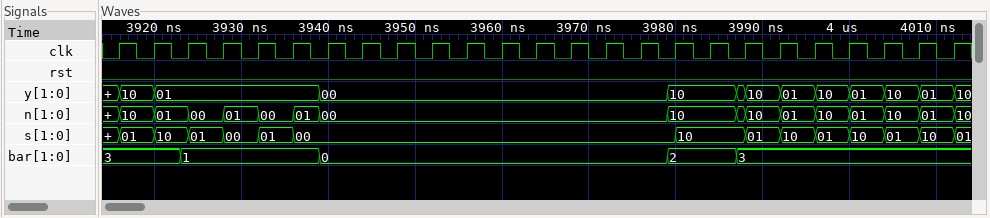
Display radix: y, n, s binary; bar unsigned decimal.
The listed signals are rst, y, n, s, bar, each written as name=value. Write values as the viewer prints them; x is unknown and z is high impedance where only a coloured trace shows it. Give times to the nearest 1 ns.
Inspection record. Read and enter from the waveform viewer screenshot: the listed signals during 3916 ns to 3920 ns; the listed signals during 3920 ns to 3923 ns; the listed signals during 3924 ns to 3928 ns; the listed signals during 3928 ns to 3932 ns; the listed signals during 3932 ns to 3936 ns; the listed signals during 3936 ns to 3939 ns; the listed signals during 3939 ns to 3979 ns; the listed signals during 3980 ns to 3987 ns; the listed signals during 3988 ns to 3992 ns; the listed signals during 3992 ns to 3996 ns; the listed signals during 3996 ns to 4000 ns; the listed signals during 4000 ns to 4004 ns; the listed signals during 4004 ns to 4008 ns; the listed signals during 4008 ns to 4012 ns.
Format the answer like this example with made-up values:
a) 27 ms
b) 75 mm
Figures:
a) rst=0, y=10, n=10, s=01, bar=3
b) rst=0, y=01, n=01, s=10, bar=3
c) rst=0, y=01, n=00, s=01, bar=1
d) rst=0, y=01, n=01, s=00, bar=1
e) rst=0, y=01, n=00, s=01, bar=1
f) rst=0, y=01, n=01, s=00, bar=1
g) rst=0, y=00, n=00, s=00, bar=0
h) rst=0, y=10, n=10, s=10, bar=2
i) rst=0, y=10, n=10, s=01, bar=3
j) rst=0, y=01, n=01, s=10, bar=3
k) rst=0, y=10, n=10, s=01, bar=3
l) rst=0, y=01, n=01, s=10, bar=3
m) rst=0, y=10, n=10, s=01, bar=3
n) rst=0, y=01, n=01, s=10, bar=3
